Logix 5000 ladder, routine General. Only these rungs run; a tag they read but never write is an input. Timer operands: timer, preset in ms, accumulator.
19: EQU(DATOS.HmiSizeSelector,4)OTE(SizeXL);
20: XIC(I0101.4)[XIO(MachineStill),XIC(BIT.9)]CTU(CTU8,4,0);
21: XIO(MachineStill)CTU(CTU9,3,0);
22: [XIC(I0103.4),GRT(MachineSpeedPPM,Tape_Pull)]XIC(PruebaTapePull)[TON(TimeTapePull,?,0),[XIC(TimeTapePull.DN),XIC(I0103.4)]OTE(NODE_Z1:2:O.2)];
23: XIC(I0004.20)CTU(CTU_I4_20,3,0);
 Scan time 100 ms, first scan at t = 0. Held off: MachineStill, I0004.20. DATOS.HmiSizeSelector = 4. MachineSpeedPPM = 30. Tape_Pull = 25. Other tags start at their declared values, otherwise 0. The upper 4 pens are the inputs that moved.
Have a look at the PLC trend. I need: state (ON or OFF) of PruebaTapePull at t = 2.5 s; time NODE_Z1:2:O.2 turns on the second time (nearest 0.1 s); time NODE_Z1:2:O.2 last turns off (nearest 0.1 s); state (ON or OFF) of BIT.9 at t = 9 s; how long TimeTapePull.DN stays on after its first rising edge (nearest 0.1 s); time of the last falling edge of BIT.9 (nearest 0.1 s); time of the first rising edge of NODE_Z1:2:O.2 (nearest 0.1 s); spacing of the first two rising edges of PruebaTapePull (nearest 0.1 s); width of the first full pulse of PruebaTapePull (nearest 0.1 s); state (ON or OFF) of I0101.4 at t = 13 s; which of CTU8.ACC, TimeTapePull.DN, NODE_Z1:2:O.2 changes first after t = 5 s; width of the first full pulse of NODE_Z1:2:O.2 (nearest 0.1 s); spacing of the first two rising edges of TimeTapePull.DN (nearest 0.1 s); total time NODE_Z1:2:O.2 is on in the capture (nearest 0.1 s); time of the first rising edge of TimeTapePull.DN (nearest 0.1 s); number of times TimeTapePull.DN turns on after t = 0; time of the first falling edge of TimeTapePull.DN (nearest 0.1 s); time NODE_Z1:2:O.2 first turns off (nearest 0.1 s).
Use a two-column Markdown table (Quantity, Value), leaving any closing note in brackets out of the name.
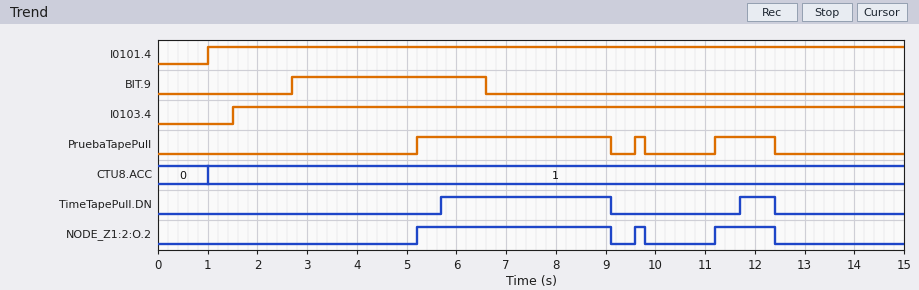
| Quantity | Value |
|---|---|
| state (ON or OFF) of PruebaTapePull at t = 2.5 s | OFF |
| time NODE_Z1:2:O.2 turns on the second time | 9.6 s |
| time NODE_Z1:2:O.2 last turns off | 12.4 s |
| state (ON or OFF) of BIT.9 at t = 9 s | OFF |
| how long TimeTapePull.DN stays on after its first rising edge | 3.4 s |
| time of the last falling edge of BIT.9 | 6.6 s |
| time of the first rising edge of NODE_Z1:2:O.2 | 5.2 s |
| spacing of the first two rising edges of PruebaTapePull | 4.4 s |
| width of the first full pulse of PruebaTapePull | 3.9 s |
| state (ON or OFF) of I0101.4 at t = 13 s | ON |
| which of CTU8.ACC, TimeTapePull.DN, NODE_Z1:2:O.2 changes first after t = 5 s | NODE_Z1:2:O.2 |
| width of the first full pulse of NODE_Z1:2:O.2 | 3.9 s |
| spacing of the first two rising edges of TimeTapePull.DN | 6.0 s |
| total time NODE_Z1:2:O.2 is on in the capture | 5.3 s |
| time of the first rising edge of TimeTapePull.DN | 5.7 s |
| number of times TimeTapePull.DN turns on after t = 0 | 2 |
| time of the first falling edge of TimeTapePull.DN | 9.1 s |
| time NODE_Z1:2:O.2 first turns off | 9.1 s |
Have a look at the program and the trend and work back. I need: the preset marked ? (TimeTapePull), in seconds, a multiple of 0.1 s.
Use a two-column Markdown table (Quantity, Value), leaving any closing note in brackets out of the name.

| Quantity | Value |
|---|---|
| the preset marked ? (TimeTapePull), in seconds, a multiple of 0.1 s | 0.5 s |
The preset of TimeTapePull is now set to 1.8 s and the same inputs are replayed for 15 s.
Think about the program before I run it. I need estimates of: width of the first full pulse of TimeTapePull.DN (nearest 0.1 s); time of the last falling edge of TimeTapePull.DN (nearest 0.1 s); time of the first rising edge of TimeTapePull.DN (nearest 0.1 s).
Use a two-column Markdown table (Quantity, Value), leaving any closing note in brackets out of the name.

| Quantity | Value |
|---|---|
| width of the first full pulse of TimeTapePull.DN | 2.1 s |
| time of the last falling edge of TimeTapePull.DN | 9.1 s |
| time of the first rising edge of TimeTapePull.DN | 7.0 s |
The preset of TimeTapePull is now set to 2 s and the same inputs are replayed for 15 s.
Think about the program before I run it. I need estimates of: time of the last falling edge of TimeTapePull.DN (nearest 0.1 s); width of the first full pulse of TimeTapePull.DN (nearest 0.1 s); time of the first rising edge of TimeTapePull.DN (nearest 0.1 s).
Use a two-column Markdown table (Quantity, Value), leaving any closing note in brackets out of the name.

| Quantity | Value |
|---|---|
| time of the last falling edge of TimeTapePull.DN | 9.1 s |
| width of the first full pulse of TimeTapePull.DN | 1.9 s |
| time of the first rising edge of TimeTapePull.DN | 7.2 s |
